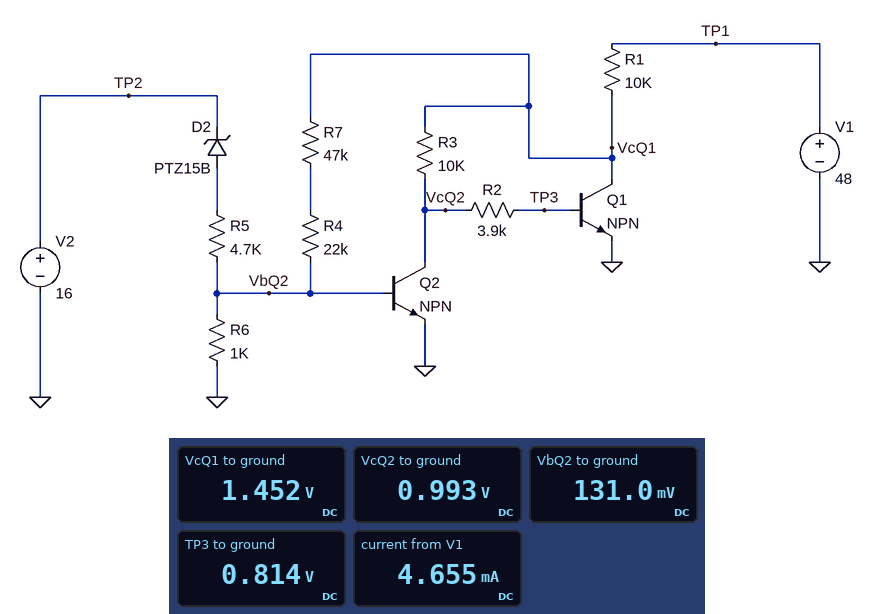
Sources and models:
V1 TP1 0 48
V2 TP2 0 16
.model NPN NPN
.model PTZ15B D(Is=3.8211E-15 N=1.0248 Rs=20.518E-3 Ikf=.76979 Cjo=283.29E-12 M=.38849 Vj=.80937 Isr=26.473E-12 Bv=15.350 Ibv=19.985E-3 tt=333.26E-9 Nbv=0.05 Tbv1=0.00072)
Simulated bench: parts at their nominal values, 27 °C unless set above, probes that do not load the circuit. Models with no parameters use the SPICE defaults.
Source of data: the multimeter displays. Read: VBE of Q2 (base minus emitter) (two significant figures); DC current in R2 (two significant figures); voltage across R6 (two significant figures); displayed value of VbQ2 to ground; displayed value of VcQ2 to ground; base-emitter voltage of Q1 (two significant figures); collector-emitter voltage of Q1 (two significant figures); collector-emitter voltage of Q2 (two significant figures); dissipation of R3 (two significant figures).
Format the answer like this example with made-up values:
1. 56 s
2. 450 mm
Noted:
1. 130 mV
2. 46 µA
3. 130 mV
4. 131.0 mV
5. 0.993 V
6. 810 mV
7. 1.5 V
8. 990 mV
9. 21 µW
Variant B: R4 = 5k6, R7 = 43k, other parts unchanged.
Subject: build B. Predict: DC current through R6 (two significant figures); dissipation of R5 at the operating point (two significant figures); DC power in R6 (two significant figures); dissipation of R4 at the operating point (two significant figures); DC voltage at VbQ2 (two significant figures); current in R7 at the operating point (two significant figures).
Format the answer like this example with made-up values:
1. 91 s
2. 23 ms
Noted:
1. 140 µA
2. 57 µW
3. 19 µW
4. 4.1 µW
5. 140 mV
6. 27 µA
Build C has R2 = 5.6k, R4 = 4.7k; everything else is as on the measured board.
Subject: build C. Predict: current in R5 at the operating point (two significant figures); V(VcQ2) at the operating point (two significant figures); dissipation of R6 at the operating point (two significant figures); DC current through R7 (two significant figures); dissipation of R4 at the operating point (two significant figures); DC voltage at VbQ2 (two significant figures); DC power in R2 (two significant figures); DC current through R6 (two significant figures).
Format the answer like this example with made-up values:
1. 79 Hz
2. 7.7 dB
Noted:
1. 110 µA
2. 1.1 V
3. 19 µW
4. 27 µA
5. 3.4 µW
6. 140 mV
7. 12 µW
8. 140 µA
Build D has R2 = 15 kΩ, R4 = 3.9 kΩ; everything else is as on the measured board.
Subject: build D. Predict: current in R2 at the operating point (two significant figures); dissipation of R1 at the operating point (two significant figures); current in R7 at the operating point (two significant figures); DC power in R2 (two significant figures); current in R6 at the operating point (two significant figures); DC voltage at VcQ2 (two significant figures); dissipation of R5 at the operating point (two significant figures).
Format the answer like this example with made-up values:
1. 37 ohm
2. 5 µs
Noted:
1. 45 µA
2. 210 mW
3. 35 µA
4. 31 µW
5. 140 µA
6. 1.5 V
7. 56 µW
